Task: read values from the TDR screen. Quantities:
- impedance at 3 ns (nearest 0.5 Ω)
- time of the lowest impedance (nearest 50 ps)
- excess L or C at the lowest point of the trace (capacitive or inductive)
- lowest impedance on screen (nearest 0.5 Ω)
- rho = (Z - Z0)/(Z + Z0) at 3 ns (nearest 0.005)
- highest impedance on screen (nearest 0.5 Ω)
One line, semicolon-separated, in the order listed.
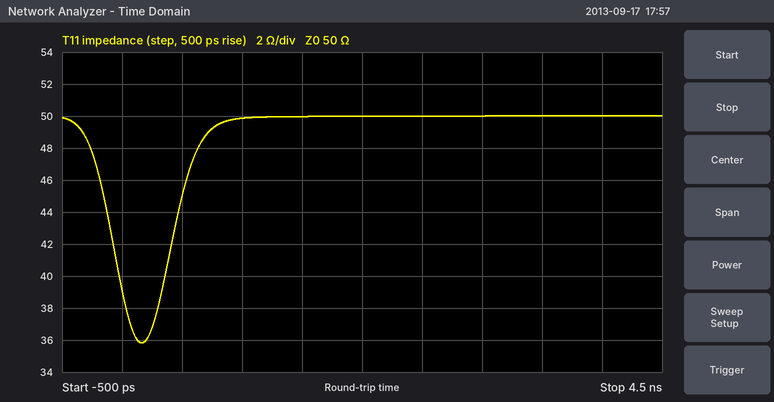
50.0 Ω; 150 ps; capacitive; 36.0 Ω; 0.000; 50.0 Ω
